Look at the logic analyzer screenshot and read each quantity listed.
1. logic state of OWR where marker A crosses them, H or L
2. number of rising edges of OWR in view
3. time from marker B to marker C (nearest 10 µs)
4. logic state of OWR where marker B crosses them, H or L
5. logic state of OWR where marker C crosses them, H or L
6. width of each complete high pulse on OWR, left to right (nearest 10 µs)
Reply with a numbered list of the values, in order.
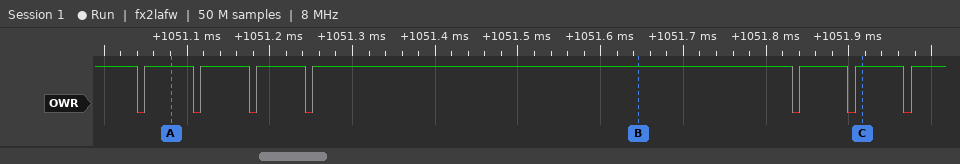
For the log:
1. OWR=H
2. 7
3. 270 µs
4. OWR=H
5. OWR=H
6. 60 µs, 60 µs, 60 µs, 580 µs, 60 µs, 60 µs
